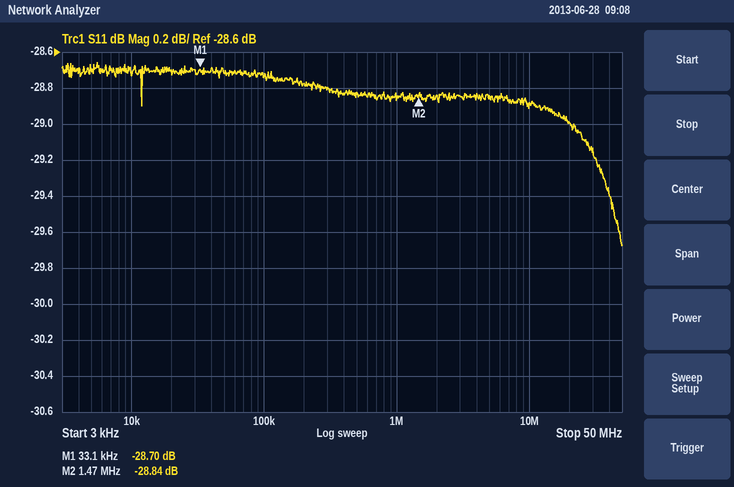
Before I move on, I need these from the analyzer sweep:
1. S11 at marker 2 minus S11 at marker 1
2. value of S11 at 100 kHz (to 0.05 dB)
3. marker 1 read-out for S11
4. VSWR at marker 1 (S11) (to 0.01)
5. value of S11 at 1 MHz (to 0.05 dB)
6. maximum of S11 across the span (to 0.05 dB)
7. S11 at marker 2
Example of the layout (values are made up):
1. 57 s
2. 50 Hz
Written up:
1. -0.14 dB
2. -28.75 dB
3. -28.70 dB
4. 1.08
5. -28.85 dB
6. -28.65 dB
7. -28.84 dB
